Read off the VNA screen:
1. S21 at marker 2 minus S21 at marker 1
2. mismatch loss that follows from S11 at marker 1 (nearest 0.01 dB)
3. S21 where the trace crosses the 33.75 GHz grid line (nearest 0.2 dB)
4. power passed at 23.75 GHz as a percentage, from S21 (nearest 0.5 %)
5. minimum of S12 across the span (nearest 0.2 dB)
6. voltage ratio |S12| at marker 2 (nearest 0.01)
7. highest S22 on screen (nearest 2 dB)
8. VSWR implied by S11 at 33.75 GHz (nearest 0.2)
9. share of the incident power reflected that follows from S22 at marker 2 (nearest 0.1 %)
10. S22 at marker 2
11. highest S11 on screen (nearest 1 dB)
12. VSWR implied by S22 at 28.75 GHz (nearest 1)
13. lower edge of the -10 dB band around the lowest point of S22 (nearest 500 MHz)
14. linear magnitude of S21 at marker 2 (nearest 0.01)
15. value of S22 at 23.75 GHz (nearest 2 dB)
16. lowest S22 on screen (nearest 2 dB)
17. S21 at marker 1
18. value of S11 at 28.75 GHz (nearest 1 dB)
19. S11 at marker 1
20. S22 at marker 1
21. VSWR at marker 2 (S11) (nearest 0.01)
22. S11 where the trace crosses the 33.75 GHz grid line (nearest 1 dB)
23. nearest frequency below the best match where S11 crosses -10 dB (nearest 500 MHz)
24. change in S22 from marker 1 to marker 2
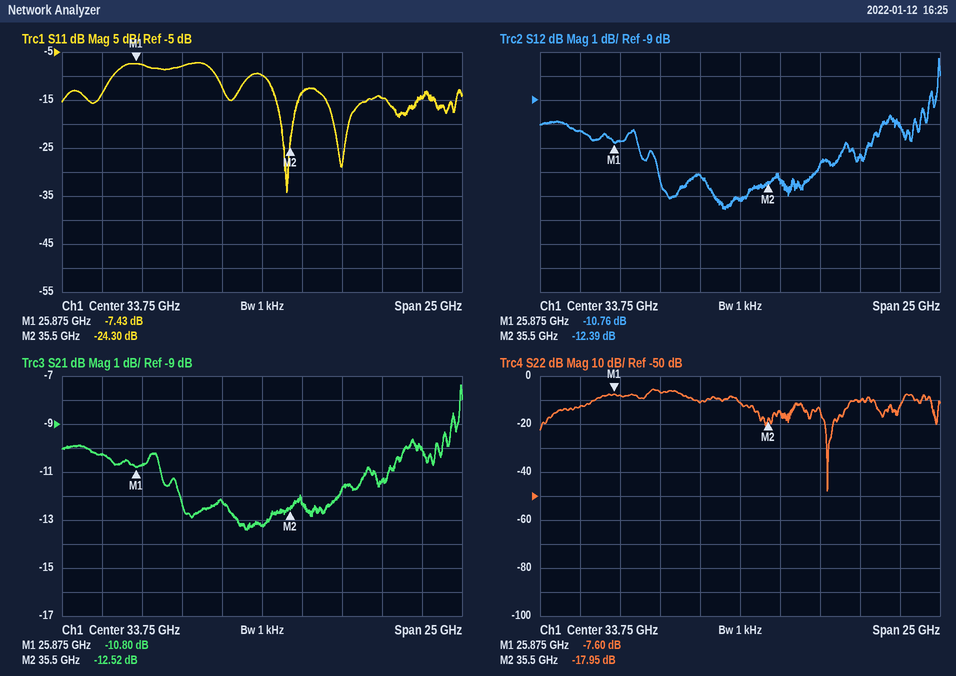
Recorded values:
-1.72 dB
0.87 dB
-13.2 dB
9.5 %
-13.6 dB
0.24
-6 dB
2.0
1.6 %
-17.95 dB
-7 dB
3
33.5 GHz
0.24
-12 dB
-48 dB
-10.80 dB
-8 dB
-7.43 dB
-7.60 dB
1.13
-10 dB
34.0 GHz
-10.35 dB
